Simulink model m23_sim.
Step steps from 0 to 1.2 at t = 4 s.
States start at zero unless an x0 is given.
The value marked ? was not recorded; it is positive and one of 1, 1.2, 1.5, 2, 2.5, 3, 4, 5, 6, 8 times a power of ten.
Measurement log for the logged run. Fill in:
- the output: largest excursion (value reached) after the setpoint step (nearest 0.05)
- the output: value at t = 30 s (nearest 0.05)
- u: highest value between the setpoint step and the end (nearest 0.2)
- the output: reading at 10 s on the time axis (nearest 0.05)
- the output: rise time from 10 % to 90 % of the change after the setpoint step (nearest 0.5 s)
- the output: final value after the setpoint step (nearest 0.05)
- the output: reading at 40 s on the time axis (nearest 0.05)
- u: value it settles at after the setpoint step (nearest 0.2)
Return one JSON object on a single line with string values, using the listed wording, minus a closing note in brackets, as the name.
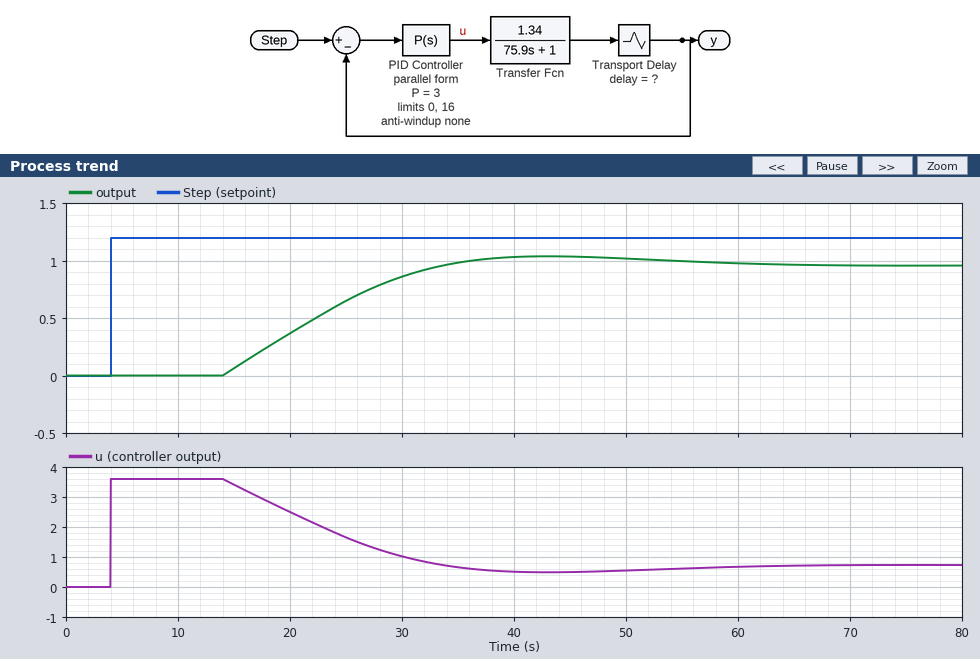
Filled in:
{"the output: largest excursion (value reached) after the setpoint step": "1.05", "the output: value at t = 30 s": "0.85", "u: highest value between the setpoint step and the end": "3.6", "the output: reading at 10 s on the time axis": "0.00", "the output: rise time from 10 % to 90 % of the change after the setpoint step": "14.5 s", "the output: final value after the setpoint step": "0.95", "the output: reading at 40 s on the time axis": "1.05", "u: value it settles at after the setpoint step": "0.8"}
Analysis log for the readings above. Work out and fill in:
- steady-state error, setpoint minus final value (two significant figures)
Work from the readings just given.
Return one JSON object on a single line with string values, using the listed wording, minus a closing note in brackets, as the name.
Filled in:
{"steady-state error, setpoint minus final value": "0.25"}
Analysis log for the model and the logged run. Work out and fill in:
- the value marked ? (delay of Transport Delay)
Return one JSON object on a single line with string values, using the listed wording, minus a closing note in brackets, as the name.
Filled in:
{"the value marked ?": "10"}
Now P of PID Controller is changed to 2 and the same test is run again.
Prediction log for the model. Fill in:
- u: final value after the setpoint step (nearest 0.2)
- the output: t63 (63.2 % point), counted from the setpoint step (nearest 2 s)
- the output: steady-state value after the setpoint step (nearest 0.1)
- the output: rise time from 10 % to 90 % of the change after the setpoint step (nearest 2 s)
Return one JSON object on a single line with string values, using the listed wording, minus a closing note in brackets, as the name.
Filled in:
{"u: final value after the setpoint step": "0.6", "the output: t63 (63.2 % point), counted from the setpoint step": "24 s", "the output: steady-state value after the setpoint step": "0.9", "the output: rise time from 10 % to 90 % of the change after the setpoint step": "26 s"}
